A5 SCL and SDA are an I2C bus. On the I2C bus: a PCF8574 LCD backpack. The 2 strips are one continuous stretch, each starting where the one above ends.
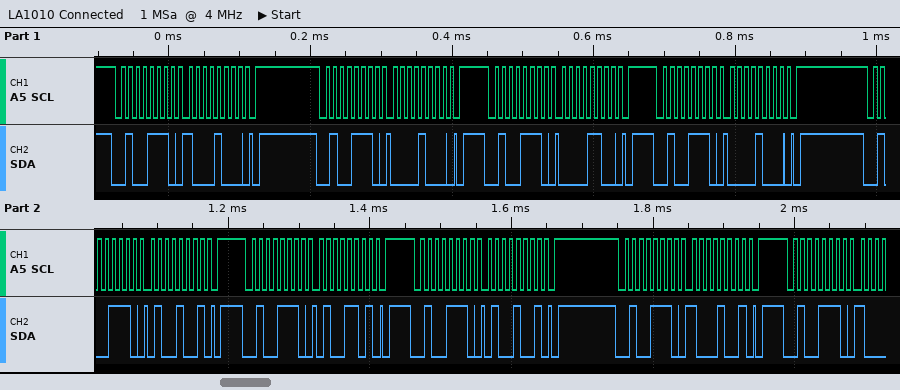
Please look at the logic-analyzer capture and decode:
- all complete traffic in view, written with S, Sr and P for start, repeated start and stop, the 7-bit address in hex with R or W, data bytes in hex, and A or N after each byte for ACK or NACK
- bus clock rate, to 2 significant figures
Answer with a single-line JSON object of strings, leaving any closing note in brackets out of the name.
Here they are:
{"all complete traffic in view, written with S, Sr and P for start, repeated start and stop, the 7-bit address in hex with R or W, data bytes in hex, and A or N after each byte for ACK or NACK": "S 27W A 88 A P S 27W A 08 A P S 27W A 0C A P S 27W A 08 A P S 27W A 49 A P S 27W A 4D A P S 27W A 49 A P S 27W A 89 A P S 27W A", "bus clock rate, to 2 significant figures": "100 kHz"}
